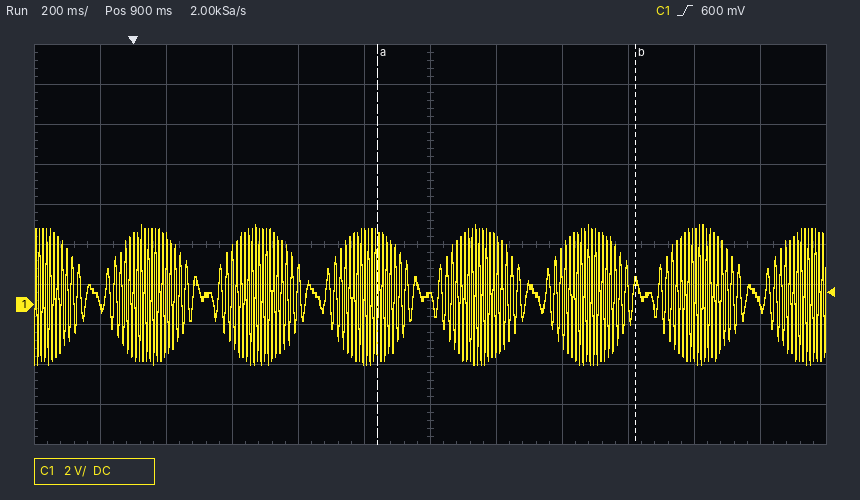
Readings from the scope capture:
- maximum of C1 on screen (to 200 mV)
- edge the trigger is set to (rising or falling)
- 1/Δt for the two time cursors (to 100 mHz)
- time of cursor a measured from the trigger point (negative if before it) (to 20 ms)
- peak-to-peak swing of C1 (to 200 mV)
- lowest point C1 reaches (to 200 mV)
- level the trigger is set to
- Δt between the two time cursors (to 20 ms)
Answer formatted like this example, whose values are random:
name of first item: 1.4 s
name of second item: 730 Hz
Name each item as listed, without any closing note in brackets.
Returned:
maximum of C1 on screen: 4.0 V
edge the trigger is set to: rising
1/Δt for the two time cursors: 1.3 Hz
time of cursor a measured from the trigger point (negative if before it): +740 ms
peak-to-peak swing of C1: 7.0 V
lowest point C1 reaches: -3.0 V
level the trigger is set to: 600 mV
Δt between the two time cursors: 780 ms
